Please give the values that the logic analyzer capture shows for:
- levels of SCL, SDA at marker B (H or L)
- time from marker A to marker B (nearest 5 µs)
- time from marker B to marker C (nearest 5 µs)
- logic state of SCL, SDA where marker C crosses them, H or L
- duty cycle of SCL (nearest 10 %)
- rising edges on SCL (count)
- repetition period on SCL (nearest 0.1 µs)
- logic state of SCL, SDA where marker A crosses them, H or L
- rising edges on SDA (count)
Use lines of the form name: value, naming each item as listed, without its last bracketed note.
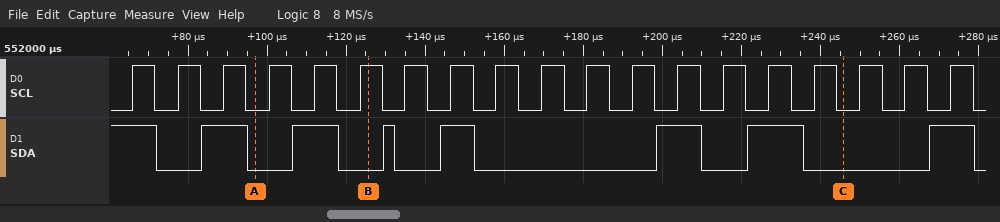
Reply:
levels of SCL, SDA at marker B: SCL=H, SDA=L
time from marker A to marker B: 30 µs
time from marker B to marker C: 120 µs
logic state of SCL, SDA where marker C crosses them, H or L: SCL=L, SDA=L
duty cycle of SCL: 50 %
rising edges on SCL: 19
repetition period on SCL: 11.5 µs
logic state of SCL, SDA where marker A crosses them, H or L: SCL=L, SDA=L
rising edges on SDA: 7
